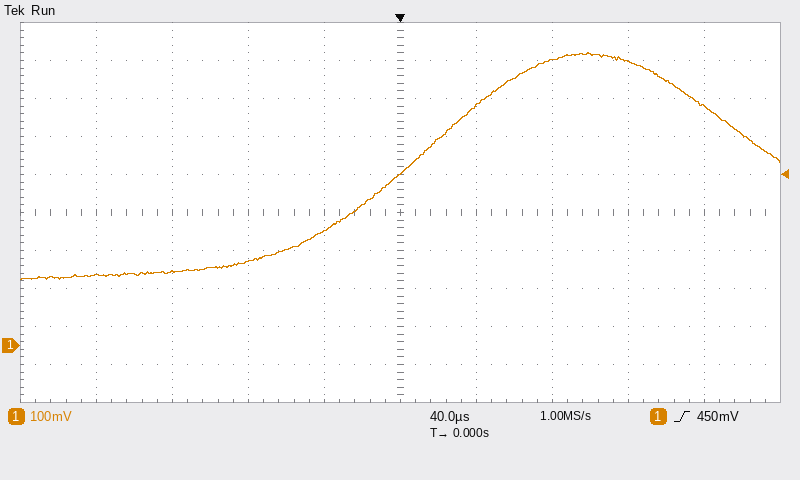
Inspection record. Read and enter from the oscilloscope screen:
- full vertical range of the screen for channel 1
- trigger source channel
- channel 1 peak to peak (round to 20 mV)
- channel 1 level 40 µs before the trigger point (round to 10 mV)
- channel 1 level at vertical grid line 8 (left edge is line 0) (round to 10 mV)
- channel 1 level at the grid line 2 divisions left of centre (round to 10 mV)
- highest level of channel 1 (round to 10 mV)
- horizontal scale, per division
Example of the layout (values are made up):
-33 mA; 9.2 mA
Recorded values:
1 V; channel 1; 600 mV; 300 mV; 750 mV; 220 mV; 770 mV; 40 µs
